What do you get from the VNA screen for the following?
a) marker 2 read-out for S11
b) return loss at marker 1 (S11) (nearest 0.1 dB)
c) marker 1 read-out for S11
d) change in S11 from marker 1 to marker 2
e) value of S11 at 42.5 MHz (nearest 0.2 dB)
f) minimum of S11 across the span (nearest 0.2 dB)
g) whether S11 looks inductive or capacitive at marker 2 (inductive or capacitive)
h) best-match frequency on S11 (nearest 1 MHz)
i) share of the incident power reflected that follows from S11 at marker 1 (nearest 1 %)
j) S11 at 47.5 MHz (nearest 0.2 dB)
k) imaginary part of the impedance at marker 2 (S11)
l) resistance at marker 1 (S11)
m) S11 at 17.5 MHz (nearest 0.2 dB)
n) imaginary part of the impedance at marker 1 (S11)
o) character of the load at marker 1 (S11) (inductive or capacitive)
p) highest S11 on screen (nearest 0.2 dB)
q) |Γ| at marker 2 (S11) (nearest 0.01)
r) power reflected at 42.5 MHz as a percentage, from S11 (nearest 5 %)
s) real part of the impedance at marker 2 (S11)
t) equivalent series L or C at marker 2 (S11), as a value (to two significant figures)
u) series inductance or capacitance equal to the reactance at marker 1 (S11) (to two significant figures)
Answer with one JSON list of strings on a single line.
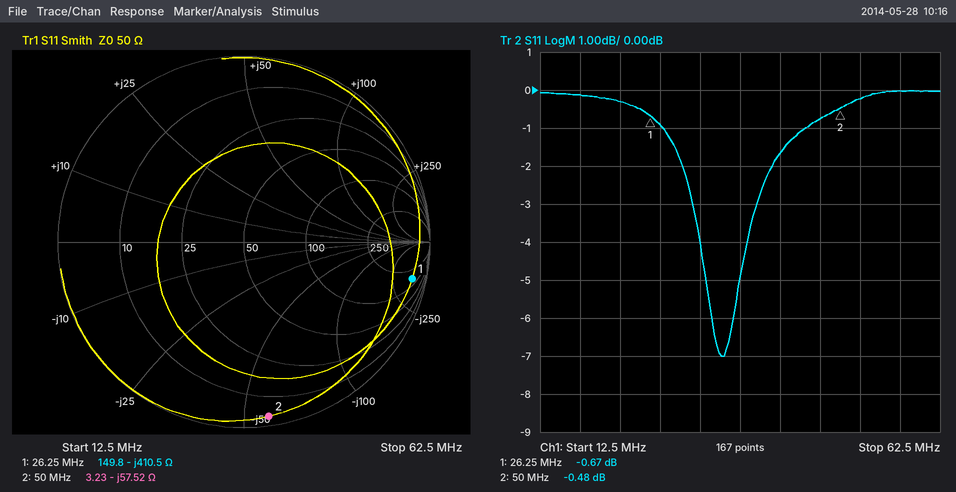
["-0.48 dB", "0.7 dB", "-0.67 dB", "0.19 dB", "-1.6 dB", "-7.0 dB", "capacitive", "35 MHz", "86 %", "-0.8 dB", "-57.52 Ω", "149.8 Ω", "-0.2 dB", "-410.5 Ω", "capacitive", "0.0 dB", "0.95", "70 %", "3.23 Ω", "55 pF", "15 pF"]
